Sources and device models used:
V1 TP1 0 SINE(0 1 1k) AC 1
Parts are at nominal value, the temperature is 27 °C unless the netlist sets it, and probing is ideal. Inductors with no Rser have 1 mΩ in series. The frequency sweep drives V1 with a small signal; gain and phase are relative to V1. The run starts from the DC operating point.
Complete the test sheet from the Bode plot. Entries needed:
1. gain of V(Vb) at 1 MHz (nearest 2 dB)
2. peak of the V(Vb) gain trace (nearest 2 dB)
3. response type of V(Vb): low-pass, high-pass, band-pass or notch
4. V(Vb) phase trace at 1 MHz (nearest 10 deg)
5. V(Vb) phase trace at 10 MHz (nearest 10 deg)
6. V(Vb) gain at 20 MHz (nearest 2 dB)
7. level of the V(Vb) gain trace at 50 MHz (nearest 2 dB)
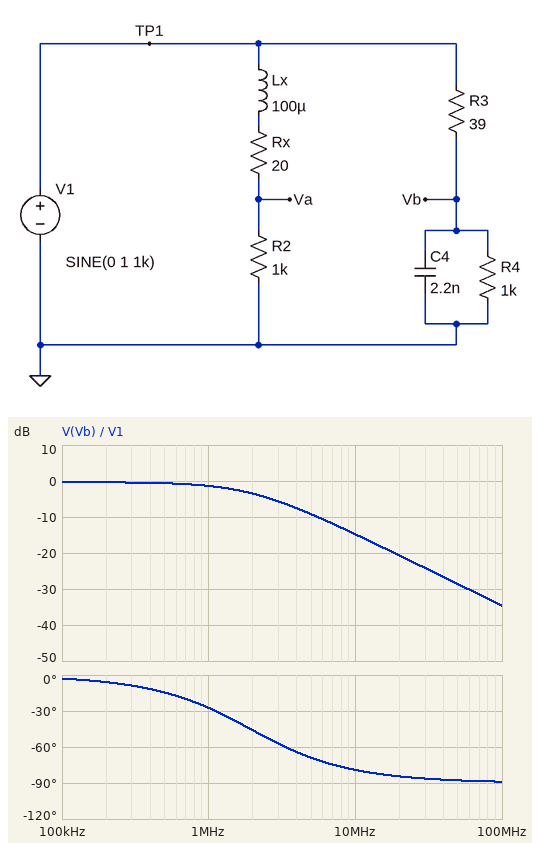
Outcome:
-2 dB
0 dB
low-pass
-30 deg
-80 deg
-20 dB
-28 dB
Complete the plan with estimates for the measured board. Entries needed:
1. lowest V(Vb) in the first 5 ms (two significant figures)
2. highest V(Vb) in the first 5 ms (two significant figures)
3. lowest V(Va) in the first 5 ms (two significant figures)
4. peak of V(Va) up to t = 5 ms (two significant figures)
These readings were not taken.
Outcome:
-960 mV
960 mV
-980 mV
980 mV
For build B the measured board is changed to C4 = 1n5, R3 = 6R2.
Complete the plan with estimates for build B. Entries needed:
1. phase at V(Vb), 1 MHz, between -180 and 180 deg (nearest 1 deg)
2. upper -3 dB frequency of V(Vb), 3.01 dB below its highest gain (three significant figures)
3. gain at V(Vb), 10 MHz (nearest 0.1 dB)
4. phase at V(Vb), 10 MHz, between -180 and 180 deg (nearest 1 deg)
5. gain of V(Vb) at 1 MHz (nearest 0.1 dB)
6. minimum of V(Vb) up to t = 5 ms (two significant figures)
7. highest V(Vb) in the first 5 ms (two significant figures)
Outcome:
-3 deg
17.2 MHz
-1.3 dB
-30 deg
-0.1 dB
-990 mV
990 mV
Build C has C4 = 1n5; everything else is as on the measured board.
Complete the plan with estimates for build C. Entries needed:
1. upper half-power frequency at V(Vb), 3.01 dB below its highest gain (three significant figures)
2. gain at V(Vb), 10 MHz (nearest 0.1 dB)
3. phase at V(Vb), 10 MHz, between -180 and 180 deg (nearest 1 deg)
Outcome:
2.83 MHz
-11.6 dB
-74 deg
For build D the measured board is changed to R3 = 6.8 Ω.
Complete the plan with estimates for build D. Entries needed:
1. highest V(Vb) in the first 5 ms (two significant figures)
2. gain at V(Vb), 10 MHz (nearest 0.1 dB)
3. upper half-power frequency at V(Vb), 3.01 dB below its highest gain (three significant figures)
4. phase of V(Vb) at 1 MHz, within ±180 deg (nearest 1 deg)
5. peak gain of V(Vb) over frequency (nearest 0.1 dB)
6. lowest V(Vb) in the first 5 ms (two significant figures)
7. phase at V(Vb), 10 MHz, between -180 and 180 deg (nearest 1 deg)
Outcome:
990 mV
-2.8 dB
10.7 MHz
-5 deg
-0.1 dB
-990 mV
-43 deg
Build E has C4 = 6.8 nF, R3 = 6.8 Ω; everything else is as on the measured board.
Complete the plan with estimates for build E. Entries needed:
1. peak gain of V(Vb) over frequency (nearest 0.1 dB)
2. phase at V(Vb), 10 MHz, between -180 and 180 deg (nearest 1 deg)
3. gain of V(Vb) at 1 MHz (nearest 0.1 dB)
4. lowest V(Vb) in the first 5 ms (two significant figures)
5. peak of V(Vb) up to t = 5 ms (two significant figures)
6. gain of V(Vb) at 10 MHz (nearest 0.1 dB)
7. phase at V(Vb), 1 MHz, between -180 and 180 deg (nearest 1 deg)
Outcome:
-0.1 dB
-71 deg
-0.4 dB
-990 mV
990 mV
-9.8 dB
-16 deg
